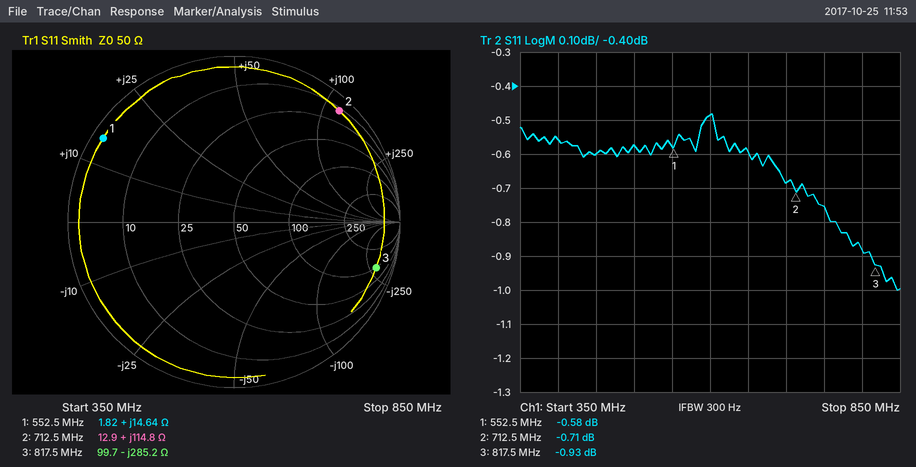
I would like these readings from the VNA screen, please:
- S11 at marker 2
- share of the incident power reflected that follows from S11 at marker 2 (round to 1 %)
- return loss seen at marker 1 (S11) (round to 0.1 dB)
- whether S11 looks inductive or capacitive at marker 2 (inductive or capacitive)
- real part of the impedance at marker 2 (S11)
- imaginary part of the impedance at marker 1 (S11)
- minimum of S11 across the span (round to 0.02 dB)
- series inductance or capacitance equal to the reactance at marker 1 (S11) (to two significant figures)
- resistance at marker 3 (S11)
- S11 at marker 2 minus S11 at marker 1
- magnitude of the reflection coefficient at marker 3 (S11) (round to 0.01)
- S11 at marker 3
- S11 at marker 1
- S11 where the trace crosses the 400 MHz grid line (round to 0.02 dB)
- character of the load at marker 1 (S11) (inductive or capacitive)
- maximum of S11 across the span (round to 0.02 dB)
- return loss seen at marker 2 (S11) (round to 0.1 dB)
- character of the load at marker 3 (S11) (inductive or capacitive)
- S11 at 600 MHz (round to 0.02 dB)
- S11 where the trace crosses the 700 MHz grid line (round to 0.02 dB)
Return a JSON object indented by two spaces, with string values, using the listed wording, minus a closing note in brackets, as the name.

{
  "S11 at marker 2": "-0.71 dB",
  "share of the incident power reflected that follows from S11 at marker 2": "85 %",
  "return loss seen at marker 1 (S11)": "0.6 dB",
  "whether S11 looks inductive or capacitive at marker 2": "inductive",
  "real part of the impedance at marker 2": "12.9 Ω",
  "imaginary part of the impedance at marker 1": "+14.64 Ω",
  "minimum of S11 across the span": "-1.00 dB",
  "series inductance or capacitance equal to the reactance at marker 1 (S11)": "4.2 nH",
  "resistance at marker 3": "99.7 Ω",
  "S11 at marker 2 minus S11 at marker 1": "-0.13 dB",
  "magnitude of the reflection coefficient at marker 3 (S11)": "0.90",
  "S11 at marker 3": "-0.93 dB",
  "S11 at marker 1": "-0.58 dB",
  "S11 where the trace crosses the 400 MHz grid line": "-0.56 dB",
  "character of the load at marker 1 (S11)": "inductive",
  "maximum of S11 across the span": "-0.48 dB",
  "return loss seen at marker 2 (S11)": "0.7 dB",
  "character of the load at marker 3 (S11)": "capacitive",
  "S11 at 600 MHz": "-0.48 dB",
  "S11 where the trace crosses the 700 MHz grid line": "-0.68 dB"
}
